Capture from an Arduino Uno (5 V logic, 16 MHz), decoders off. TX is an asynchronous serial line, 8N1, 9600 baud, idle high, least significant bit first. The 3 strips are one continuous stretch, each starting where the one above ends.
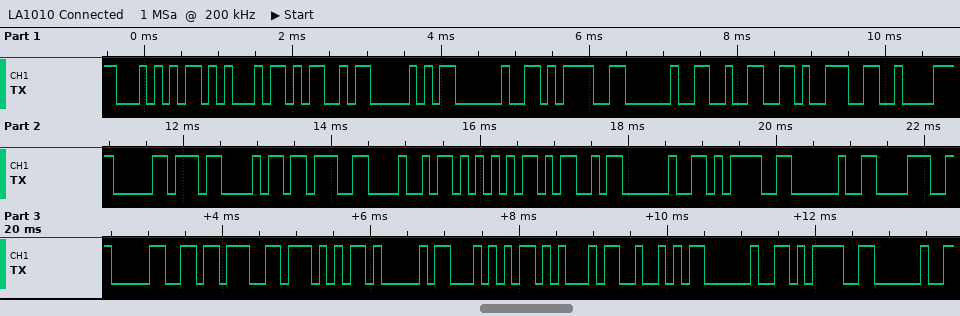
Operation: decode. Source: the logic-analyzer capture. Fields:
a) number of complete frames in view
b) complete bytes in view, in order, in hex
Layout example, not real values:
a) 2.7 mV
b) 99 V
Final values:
a) 30
b) 54 45 4D 50 20 3D 20 32 39 C2 B0 43 3B 48 55 4D 20 3D 20 38 30 3B 57 41 54 45 52 20 3D 20
